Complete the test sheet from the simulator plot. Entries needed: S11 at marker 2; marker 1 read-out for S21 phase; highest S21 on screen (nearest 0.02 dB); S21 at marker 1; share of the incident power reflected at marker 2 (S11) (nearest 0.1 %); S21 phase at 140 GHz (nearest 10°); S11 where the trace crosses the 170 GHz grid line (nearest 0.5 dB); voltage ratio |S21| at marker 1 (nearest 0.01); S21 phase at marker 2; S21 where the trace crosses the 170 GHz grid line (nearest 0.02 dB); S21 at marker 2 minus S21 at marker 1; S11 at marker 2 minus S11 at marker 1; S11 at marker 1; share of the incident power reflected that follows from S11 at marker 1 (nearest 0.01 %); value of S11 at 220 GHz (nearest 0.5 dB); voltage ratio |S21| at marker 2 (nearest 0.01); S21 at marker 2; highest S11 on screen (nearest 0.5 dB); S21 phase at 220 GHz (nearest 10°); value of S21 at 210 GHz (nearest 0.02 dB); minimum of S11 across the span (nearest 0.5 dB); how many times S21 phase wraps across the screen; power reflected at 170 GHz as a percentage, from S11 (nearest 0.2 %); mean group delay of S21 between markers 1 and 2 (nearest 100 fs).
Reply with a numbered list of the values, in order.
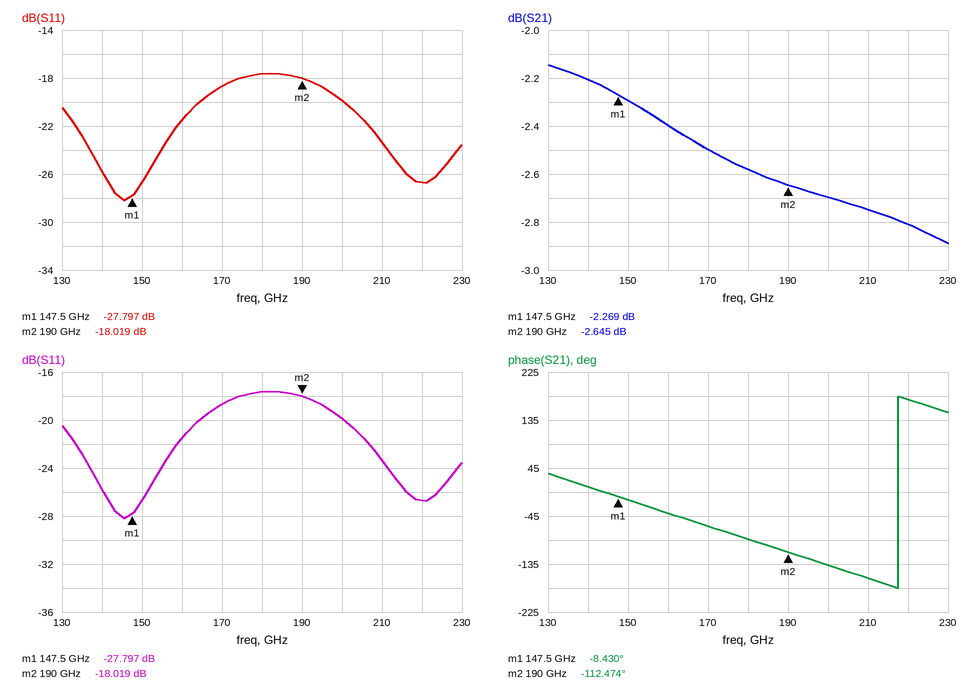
1. -18.019 dB
2. -8.430°
3. -2.14 dB
4. -2.269 dB
5. 1.6 %
6. 10°
7. -18.5 dB
8. 0.77
9. -112.474°
10. -2.50 dB
11. -0.376 dB
12. 9.778 dB
13. -27.797 dB
14. 0.17 %
15. -26.5 dB
16. 0.74
17. -2.645 dB
18. -17.5 dB
19. 170°
20. -2.74 dB
21. -28.0 dB
22. 1
23. 1.4 %
24. 6.8 ps
